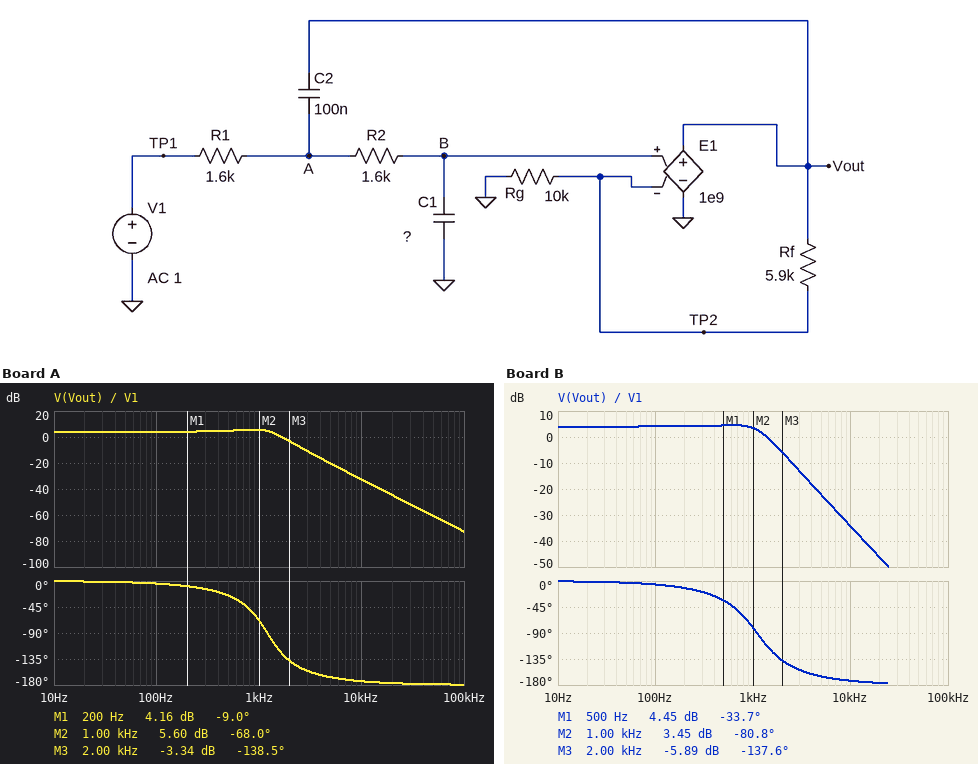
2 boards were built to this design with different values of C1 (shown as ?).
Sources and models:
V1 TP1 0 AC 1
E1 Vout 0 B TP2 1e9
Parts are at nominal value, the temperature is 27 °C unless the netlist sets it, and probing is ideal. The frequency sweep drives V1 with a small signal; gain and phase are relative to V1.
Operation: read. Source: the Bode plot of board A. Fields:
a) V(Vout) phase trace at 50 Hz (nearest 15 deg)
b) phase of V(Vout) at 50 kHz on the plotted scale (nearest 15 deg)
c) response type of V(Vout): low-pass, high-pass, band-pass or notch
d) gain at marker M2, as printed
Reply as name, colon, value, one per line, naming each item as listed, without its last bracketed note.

V(Vout) phase trace at 50 Hz: 0 deg
phase of V(Vout) at 50 kHz on the plotted scale: -180 deg
response type of V(Vout): low-pass, high-pass, band-pass or notch: low-pass
gain at marker M2, as printed: 5.60 dB
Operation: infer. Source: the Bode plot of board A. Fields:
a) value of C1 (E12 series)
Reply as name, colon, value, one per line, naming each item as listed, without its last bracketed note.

value of C1: 68 nF
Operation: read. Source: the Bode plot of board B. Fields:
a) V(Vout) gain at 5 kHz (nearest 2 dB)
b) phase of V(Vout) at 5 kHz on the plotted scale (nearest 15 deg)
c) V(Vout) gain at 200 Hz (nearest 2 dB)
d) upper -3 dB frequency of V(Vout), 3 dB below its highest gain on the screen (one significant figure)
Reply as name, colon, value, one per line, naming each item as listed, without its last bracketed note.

V(Vout) gain at 5 kHz: -22 dB
phase of V(Vout) at 5 kHz on the plotted scale: -165 deg
V(Vout) gain at 200 Hz: 4 dB
upper -3 dB frequency of V(Vout), 3 dB below its highest gain on the screen: 1 kHz
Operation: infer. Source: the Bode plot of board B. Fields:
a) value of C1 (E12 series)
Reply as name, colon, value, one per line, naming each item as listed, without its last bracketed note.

value of C1: 82 nF
